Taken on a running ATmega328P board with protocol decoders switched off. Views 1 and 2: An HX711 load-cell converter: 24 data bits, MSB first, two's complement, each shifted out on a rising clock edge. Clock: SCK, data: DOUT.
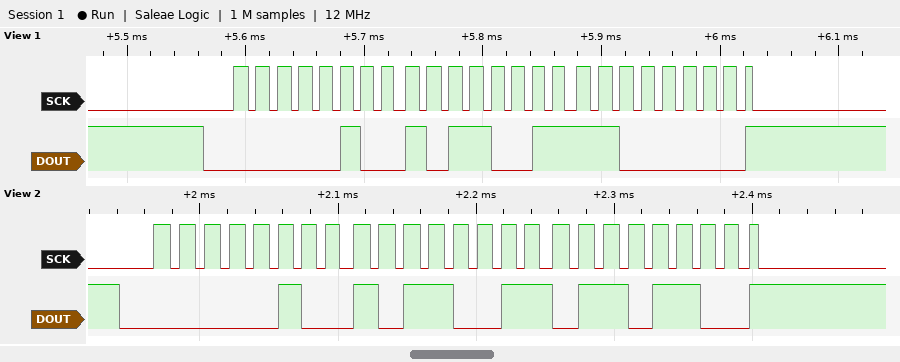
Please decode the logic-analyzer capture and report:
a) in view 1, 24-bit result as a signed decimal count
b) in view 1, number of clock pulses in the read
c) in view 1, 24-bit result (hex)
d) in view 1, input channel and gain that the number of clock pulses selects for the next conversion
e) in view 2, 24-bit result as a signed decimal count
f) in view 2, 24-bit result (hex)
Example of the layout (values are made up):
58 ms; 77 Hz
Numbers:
308160; 25; 0x04B3C0; channel A, gain 128; 308076; 0x04B36C
